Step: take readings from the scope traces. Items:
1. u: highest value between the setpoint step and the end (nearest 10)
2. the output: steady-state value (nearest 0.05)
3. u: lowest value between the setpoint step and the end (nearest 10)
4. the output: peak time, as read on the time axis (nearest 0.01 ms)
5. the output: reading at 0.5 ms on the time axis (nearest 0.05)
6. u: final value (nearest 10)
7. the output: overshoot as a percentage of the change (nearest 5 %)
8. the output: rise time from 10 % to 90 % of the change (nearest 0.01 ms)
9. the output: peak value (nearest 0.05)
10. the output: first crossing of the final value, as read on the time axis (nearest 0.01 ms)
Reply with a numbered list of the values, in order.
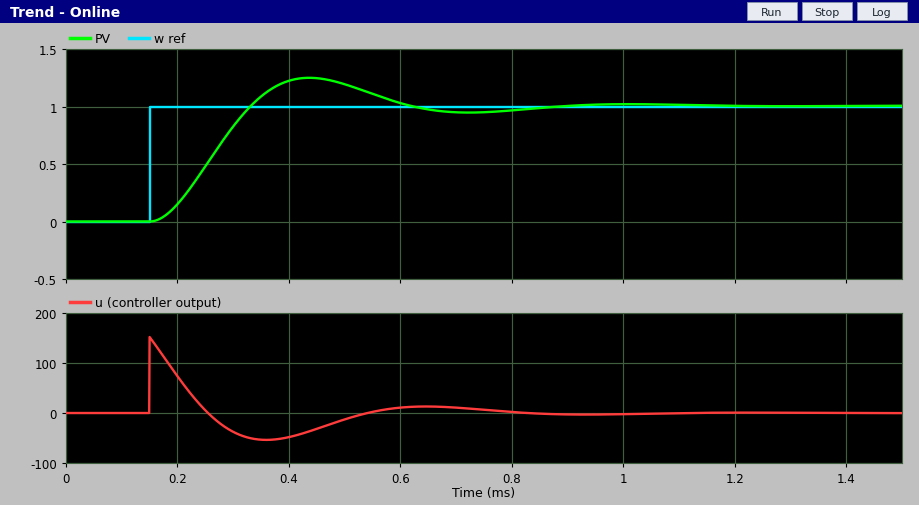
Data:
1. 150
2. 1.00
3. -50
4. 0.44 ms
5. 1.20
6. 0
7. 25 %
8. 0.12 ms
9. 1.25
10. 0.33 ms
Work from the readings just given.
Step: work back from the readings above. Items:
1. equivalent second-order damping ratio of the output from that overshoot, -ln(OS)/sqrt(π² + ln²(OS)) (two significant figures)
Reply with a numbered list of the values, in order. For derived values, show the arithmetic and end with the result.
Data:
1. ln(0.25) = -1.386; 1.386 / sqrt(9.870 + 1.922) = 0.40
